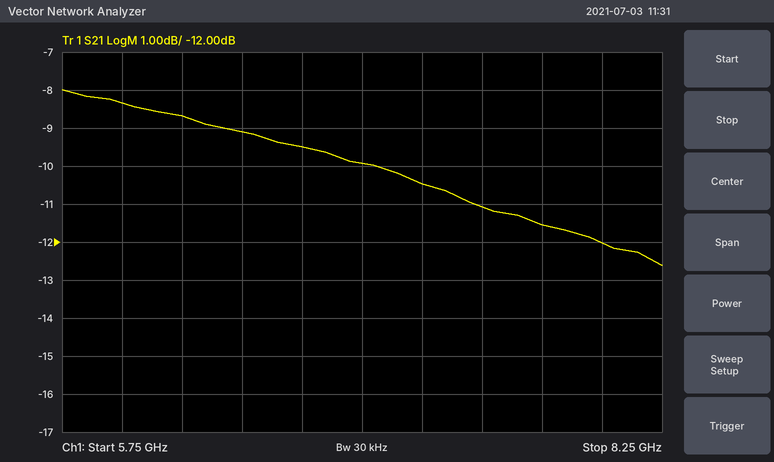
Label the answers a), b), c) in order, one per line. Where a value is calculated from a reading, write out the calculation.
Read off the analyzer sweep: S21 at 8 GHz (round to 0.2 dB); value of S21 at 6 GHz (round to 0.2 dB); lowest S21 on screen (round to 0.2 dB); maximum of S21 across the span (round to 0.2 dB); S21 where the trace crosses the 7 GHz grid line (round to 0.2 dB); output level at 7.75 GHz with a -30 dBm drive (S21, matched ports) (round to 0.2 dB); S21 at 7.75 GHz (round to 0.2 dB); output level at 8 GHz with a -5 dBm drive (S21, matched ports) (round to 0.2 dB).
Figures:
a) -12.0 dB
b) -8.4 dB
c) -12.6 dB
d) -8.0 dB
e) -10.0 dB
f) -30 dBm + (-11.6 dB) = -41.6 dBm
g) -11.6 dB
h) -5 dBm + (-12.0 dB) = -17.0 dBm
